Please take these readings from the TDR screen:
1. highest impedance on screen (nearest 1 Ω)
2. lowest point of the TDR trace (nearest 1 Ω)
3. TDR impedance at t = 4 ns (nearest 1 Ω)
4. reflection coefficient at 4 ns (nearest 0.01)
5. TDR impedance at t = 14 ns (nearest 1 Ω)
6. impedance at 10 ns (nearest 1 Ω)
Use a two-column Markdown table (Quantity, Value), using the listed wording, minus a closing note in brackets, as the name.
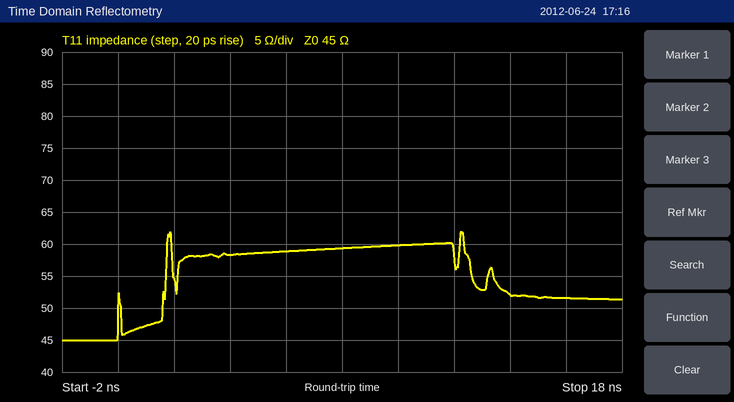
| Quantity | Value |
|---|---|
| highest impedance on screen | 62 Ω |
| lowest point of the TDR trace | 45 Ω |
| TDR impedance at t = 4 ns | 58 Ω |
| reflection coefficient at 4 ns | +0.13 |
| TDR impedance at t = 14 ns | 52 Ω |
| impedance at 10 ns | 60 Ω |
